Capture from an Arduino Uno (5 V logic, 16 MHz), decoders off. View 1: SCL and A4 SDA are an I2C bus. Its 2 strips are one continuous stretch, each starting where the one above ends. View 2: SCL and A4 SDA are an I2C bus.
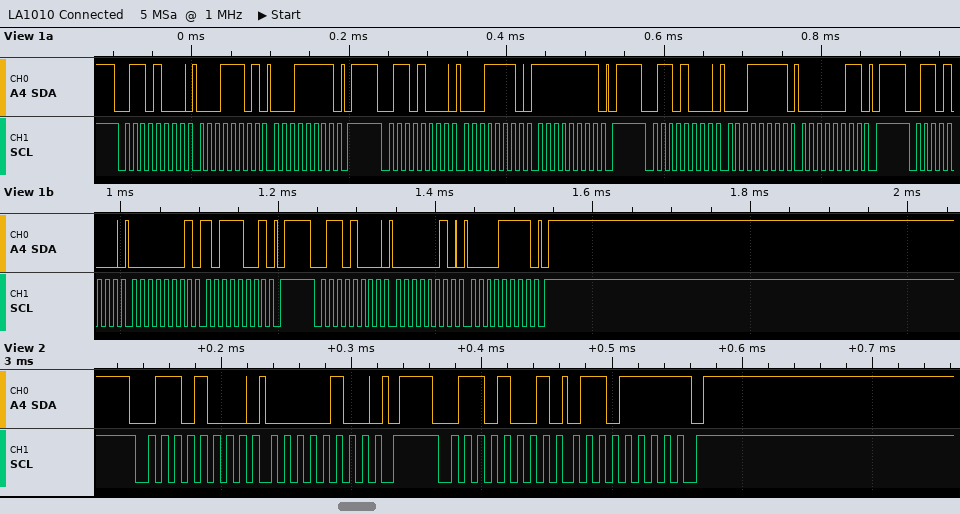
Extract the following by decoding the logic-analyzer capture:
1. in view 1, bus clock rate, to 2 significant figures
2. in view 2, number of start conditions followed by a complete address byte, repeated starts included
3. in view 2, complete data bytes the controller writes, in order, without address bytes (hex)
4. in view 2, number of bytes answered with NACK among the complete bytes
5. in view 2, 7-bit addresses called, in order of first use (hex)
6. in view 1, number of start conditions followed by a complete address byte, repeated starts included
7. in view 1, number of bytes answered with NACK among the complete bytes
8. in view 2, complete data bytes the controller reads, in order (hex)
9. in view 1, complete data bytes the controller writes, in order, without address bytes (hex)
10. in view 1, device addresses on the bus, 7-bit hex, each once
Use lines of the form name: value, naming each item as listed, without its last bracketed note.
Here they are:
in view 1, bus clock rate, to 2 significant figures: 100 kHz
in view 2, number of start conditions followed by a complete address byte, repeated starts included: 2
in view 2, complete data bytes the controller writes, in order, without address bytes: 04
in view 2, number of bytes answered with NACK among the complete bytes: 1
in view 2, 7-bit addresses called, in order of first use: 0x34
in view 1, number of start conditions followed by a complete address byte, repeated starts included: 5
in view 1, number of bytes answered with NACK among the complete bytes: 0
in view 2, complete data bytes the controller reads, in order: 6F
in view 1, complete data bytes the controller writes, in order, without address bytes: 1D 1F 1E FF 1F 03 01 B9 02 0F
in view 1, device addresses on the bus, 7-bit hex, each once: 0x34
